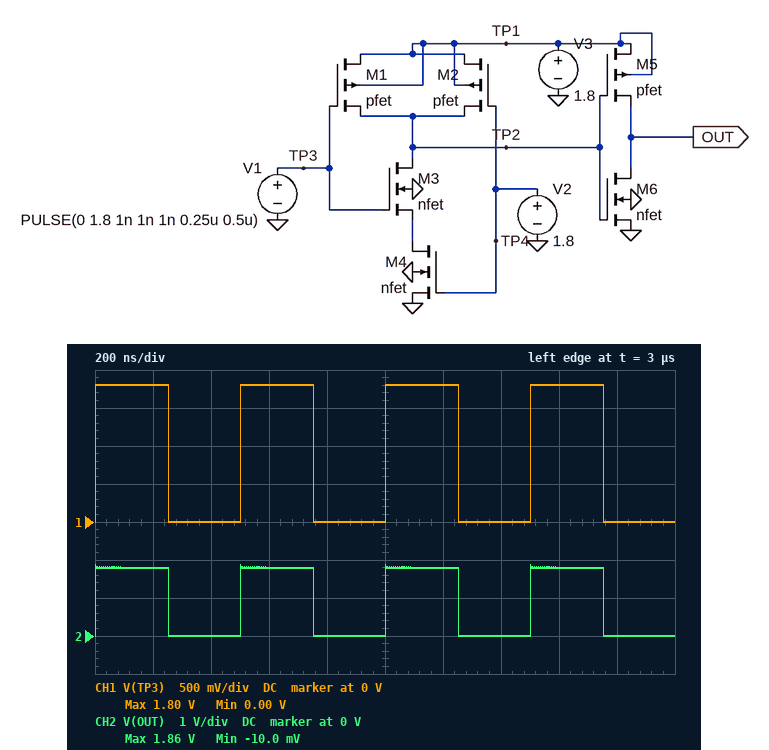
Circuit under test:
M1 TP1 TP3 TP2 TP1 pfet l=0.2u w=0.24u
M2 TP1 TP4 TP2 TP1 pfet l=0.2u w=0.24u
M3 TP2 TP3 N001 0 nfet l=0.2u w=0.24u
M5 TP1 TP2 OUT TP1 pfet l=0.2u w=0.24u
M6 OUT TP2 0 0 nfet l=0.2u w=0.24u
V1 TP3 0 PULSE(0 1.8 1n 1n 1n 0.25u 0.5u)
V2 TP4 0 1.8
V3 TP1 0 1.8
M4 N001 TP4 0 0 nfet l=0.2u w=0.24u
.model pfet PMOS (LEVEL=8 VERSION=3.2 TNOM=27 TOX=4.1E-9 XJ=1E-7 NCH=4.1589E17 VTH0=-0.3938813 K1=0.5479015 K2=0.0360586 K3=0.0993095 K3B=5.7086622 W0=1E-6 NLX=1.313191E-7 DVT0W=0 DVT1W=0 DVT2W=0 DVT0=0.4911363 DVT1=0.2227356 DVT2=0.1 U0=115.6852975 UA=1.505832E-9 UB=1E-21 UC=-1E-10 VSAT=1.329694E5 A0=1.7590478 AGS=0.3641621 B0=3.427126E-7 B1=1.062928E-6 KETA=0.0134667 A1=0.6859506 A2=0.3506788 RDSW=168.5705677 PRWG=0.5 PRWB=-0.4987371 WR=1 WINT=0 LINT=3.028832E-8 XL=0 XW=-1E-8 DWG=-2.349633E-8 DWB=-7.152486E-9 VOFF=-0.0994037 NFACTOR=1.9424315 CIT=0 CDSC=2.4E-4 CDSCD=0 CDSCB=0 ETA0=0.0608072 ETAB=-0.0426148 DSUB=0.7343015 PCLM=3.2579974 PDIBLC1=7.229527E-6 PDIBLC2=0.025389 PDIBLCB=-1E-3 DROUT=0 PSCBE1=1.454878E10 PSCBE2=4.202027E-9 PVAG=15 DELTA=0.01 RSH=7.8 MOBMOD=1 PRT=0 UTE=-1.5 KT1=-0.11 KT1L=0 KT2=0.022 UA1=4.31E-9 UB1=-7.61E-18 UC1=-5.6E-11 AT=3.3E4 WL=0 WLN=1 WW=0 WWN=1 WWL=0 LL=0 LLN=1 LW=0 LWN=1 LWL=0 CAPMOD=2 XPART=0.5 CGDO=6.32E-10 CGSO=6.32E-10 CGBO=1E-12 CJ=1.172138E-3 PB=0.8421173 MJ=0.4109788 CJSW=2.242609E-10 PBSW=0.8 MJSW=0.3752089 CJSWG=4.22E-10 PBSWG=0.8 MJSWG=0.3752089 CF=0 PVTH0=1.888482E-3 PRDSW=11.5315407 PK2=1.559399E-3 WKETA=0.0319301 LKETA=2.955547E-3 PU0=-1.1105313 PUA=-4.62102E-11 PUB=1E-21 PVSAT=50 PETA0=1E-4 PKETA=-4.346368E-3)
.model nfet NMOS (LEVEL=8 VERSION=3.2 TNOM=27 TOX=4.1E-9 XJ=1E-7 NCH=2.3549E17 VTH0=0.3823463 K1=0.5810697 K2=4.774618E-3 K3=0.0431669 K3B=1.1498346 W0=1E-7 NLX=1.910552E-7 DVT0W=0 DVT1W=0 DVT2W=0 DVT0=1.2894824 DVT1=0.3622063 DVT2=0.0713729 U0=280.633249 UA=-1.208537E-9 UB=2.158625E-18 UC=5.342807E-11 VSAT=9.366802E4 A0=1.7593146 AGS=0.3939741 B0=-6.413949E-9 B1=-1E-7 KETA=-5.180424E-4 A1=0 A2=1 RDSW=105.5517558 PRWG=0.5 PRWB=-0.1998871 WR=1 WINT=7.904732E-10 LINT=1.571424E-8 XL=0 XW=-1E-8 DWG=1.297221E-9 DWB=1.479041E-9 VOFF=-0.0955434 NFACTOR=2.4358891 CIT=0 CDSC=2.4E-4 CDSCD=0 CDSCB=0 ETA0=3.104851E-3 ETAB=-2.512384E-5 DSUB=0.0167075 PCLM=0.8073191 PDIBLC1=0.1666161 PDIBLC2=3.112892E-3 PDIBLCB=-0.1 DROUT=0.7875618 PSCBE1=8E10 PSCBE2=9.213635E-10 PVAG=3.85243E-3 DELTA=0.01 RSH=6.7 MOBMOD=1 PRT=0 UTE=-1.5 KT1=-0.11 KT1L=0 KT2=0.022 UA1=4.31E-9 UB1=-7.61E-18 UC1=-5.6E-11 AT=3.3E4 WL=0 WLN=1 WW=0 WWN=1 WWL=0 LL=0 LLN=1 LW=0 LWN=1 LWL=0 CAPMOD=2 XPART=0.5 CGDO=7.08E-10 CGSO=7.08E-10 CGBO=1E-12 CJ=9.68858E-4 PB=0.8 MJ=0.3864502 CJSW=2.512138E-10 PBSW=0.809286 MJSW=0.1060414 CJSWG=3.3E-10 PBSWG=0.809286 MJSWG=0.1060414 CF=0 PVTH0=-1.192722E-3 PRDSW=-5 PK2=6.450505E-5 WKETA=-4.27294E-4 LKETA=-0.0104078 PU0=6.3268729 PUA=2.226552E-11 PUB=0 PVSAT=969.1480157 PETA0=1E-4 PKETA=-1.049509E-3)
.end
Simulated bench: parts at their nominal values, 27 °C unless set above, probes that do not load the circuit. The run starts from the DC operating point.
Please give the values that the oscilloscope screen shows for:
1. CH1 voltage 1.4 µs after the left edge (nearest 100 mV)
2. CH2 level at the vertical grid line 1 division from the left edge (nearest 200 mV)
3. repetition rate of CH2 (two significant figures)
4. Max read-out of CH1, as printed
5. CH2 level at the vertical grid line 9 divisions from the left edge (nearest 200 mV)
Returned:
0 V
1.8 V
2.0 MHz
1.80 V
0 V
